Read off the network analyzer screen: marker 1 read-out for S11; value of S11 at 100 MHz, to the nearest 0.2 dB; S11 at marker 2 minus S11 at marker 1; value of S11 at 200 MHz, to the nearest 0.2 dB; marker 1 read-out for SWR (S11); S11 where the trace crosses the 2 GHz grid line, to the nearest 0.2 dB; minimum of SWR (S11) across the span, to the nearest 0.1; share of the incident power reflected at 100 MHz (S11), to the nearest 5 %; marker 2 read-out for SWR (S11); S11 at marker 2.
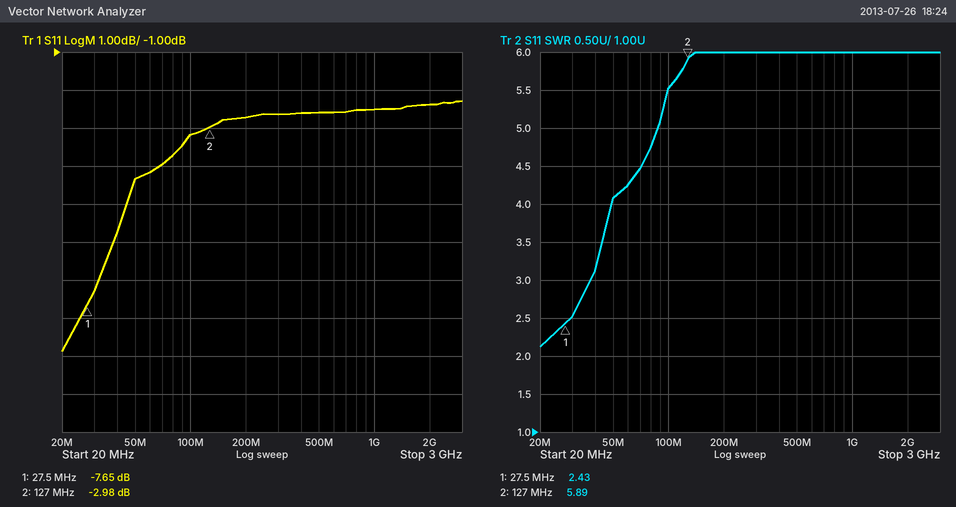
-7.65 dB
-3.2 dB
4.67 dB
-2.8 dB
2.43
-2.4 dB
2.1
50 %
5.89
-2.98 dB
